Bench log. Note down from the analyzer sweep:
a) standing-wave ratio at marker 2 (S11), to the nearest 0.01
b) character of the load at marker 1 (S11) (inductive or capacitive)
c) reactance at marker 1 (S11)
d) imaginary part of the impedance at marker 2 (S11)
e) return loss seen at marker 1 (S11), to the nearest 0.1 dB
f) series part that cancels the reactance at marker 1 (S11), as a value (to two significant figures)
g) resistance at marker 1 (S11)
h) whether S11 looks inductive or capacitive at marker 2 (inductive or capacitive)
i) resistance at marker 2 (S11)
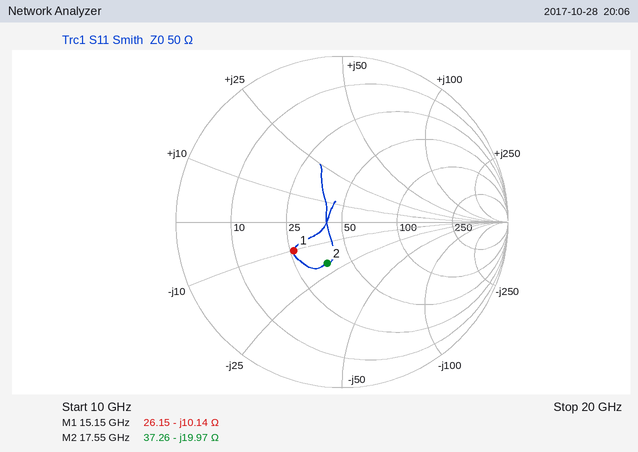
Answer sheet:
1.72
capacitive
-10.14 Ω
-19.97 Ω
9.4 dB
110 pH
26.15 Ω
capacitive
37.26 Ω
